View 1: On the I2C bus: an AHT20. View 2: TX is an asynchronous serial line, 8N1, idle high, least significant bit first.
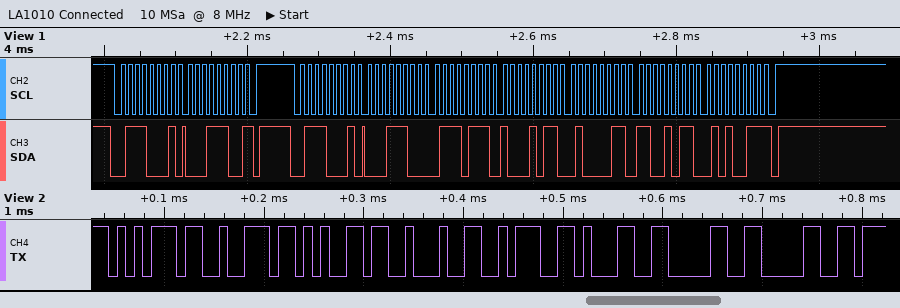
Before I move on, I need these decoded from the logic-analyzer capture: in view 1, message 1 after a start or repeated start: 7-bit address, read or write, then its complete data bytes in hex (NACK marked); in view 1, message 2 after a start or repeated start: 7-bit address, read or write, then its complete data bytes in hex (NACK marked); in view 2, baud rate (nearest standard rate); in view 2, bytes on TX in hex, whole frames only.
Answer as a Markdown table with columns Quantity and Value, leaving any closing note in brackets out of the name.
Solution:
| Quantity | Value |
|---|---|
| in view 1, message 1 after a start or repeated start: 7-bit address, read or write, then its complete data bytes in hex | 0x38 read: 1C NACK |
| in view 1, message 2 after a start or repeated start: 7-bit address, read or write, then its complete data bytes in hex | 0x38 read: 1C 77 8B 43 CB 53 NACK |
| in view 2, baud rate | 115200 baud |
| in view 2, bytes on TX in hex, whole frames only | 75 72 65 22 3A 31 30 30 |
